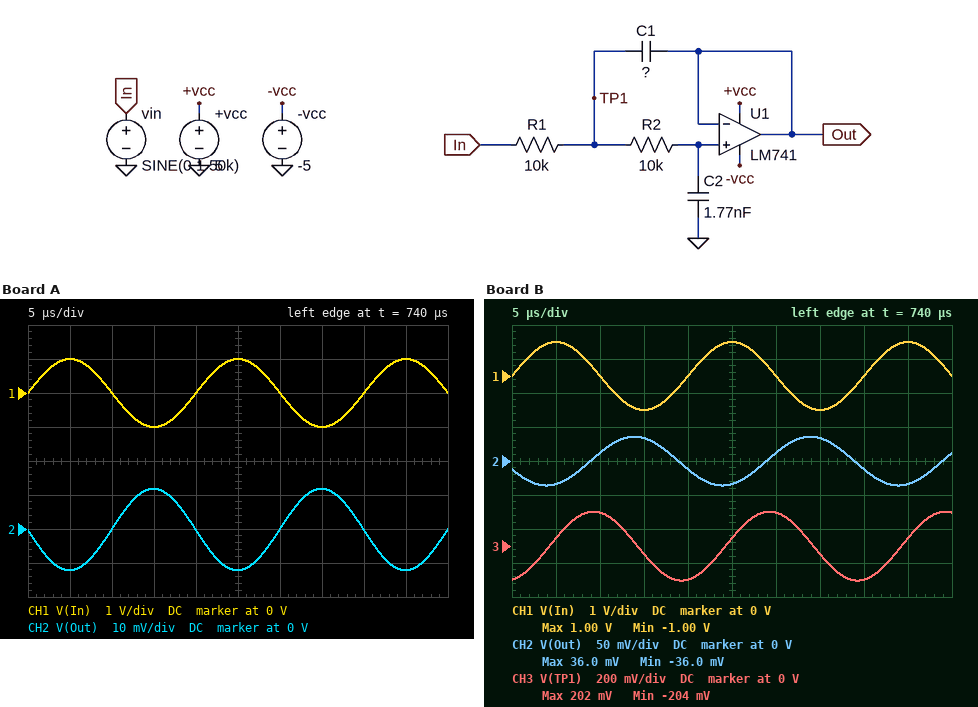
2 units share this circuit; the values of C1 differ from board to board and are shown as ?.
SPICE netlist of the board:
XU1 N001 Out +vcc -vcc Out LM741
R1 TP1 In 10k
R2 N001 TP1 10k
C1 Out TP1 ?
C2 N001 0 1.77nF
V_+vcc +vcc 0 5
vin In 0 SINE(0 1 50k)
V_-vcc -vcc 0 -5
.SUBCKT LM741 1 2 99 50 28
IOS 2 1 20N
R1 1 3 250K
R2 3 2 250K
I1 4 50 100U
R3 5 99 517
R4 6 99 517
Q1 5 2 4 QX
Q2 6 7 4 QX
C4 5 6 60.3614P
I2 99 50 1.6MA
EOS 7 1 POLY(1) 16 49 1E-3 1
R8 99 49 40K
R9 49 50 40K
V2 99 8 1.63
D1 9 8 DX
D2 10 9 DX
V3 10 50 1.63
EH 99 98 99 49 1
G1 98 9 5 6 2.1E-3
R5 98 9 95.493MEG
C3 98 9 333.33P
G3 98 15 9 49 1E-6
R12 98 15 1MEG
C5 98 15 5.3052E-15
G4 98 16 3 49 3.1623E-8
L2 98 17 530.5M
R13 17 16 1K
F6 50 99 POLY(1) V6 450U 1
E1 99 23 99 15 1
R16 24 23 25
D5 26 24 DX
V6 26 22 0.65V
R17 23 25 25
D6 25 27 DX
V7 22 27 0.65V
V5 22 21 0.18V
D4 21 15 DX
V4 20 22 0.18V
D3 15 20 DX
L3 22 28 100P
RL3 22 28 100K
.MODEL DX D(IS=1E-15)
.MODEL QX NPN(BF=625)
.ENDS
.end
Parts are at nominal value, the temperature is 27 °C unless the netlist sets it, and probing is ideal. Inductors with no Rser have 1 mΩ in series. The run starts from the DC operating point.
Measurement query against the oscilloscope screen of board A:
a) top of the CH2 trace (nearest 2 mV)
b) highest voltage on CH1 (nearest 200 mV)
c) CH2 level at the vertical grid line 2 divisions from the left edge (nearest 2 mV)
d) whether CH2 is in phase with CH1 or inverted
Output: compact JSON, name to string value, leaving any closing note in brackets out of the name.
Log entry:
{"top of the CH2 trace": "12 mV", "highest voltage on CH1": "1.0 V", "CH2 level at the vertical grid line 2 divisions from the left edge": "0 V", "whether CH2 is in phase with CH1 or inverted": "inverted"}
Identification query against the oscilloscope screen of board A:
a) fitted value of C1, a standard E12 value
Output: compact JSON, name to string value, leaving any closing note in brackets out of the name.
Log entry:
{"fitted value of C1, a standard E12 value": "4.7 nF"}
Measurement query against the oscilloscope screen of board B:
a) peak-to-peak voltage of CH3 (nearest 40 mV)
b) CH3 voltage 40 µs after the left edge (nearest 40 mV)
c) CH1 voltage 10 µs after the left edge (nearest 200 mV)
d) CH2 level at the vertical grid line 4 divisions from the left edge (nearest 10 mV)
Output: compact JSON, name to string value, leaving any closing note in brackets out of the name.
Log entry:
{"peak-to-peak voltage of CH3": "400 mV", "CH3 voltage 40 µs after the left edge": "-200 mV", "CH1 voltage 10 µs after the left edge": "0 V", "CH2 level at the vertical grid line 4 divisions from the left edge": "-10 mV"}
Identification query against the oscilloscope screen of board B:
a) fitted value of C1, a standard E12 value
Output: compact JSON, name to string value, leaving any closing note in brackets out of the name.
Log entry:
{"fitted value of C1, a standard E12 value": "1.5 nF"}
